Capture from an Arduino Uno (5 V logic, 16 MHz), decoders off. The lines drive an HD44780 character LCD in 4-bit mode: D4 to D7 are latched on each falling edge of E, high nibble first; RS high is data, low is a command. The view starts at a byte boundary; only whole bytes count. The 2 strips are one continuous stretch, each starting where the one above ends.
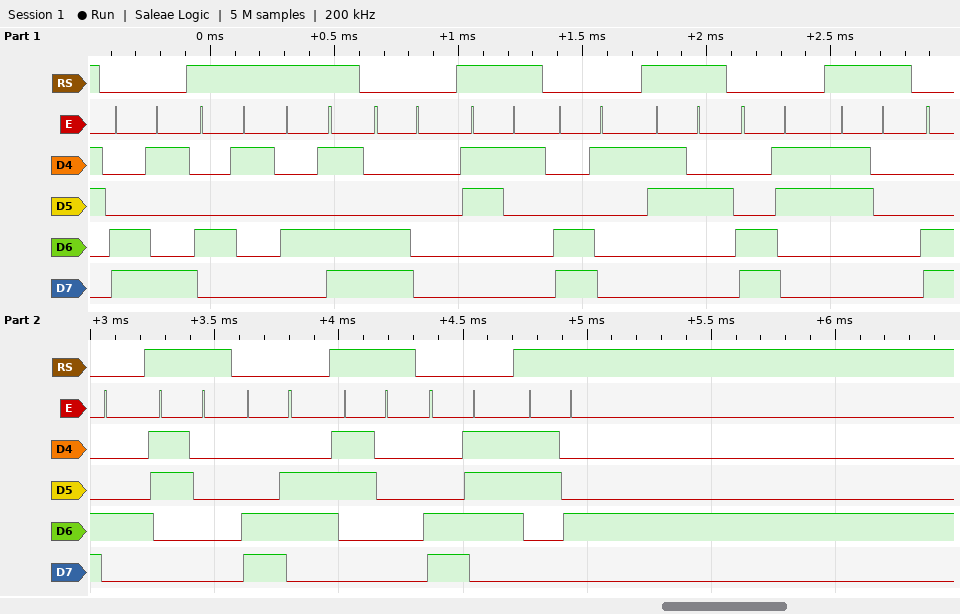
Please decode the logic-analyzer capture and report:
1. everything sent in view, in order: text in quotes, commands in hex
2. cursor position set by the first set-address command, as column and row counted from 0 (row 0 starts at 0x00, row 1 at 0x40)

0xC9 "AM" 0xC0 "1" 0xC1 "2" 0xC3 "0" 0xC4 "0" 0xC6 "0" 0xC7 "4"
column 9, row 1
